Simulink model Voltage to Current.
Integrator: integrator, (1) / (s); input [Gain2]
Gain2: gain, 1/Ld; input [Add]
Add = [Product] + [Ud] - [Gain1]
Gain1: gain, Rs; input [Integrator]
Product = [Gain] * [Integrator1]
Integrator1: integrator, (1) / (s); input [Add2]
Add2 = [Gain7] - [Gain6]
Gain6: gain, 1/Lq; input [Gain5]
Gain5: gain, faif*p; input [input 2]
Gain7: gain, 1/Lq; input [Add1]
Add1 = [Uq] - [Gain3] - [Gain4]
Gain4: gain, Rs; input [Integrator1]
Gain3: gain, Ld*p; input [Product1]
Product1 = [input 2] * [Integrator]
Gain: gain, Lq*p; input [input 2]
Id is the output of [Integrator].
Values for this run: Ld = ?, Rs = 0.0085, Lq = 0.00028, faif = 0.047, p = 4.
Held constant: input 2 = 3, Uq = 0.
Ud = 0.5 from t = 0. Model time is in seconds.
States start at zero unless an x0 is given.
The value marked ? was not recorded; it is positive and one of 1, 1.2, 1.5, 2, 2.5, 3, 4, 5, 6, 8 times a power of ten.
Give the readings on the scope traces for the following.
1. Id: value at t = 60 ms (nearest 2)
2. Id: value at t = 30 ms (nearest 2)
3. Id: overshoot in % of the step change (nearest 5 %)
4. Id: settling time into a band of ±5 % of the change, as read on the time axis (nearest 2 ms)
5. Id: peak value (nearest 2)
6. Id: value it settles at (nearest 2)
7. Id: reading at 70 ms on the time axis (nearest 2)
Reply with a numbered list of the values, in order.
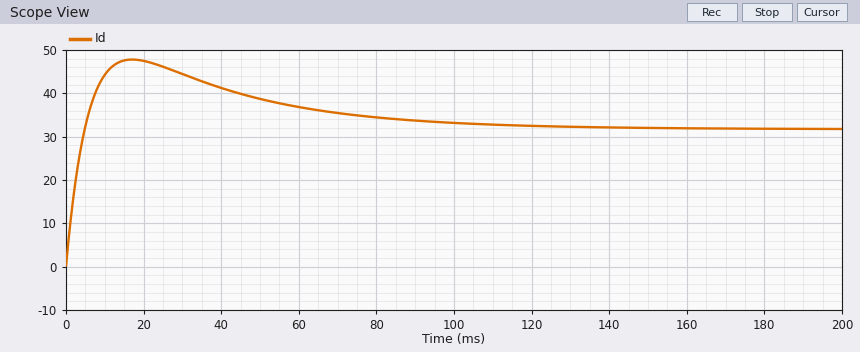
1. 36
2. 44
3. 50 %
4. 98 ms
5. 48
6. 32
7. 36
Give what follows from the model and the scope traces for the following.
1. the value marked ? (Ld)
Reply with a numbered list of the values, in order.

1. 5e-05
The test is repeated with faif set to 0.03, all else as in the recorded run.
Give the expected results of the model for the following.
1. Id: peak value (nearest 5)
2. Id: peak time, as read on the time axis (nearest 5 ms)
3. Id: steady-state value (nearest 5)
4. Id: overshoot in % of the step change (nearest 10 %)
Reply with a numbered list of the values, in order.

1. 50
2. 20 ms
3. 40
4. 20 %
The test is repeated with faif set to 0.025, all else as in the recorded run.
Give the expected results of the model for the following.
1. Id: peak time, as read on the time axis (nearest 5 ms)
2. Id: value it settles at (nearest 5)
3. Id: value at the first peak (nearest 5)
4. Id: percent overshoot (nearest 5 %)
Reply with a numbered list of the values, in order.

1. 20 ms
2. 45
3. 50
4. 20 %
